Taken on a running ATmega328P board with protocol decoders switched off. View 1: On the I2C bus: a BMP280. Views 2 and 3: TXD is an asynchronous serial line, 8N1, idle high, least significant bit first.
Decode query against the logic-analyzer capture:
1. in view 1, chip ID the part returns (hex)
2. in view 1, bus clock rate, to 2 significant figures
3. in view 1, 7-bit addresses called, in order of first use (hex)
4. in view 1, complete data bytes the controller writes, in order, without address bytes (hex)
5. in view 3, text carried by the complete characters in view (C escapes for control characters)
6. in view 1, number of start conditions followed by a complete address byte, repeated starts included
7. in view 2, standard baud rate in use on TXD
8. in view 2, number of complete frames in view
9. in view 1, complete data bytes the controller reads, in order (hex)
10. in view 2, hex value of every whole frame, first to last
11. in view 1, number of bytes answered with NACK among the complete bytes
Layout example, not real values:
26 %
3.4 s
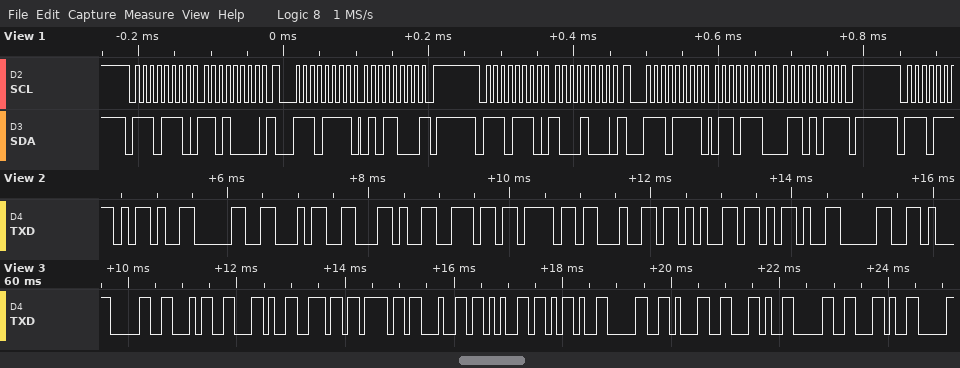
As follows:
0x58
100 kHz
0x77
D0 88
"04,node-01,0,"
4
9600 baud
10
58 6E 6B
2D 30 34 2C 6E 6F 64 65 2D 30
2
